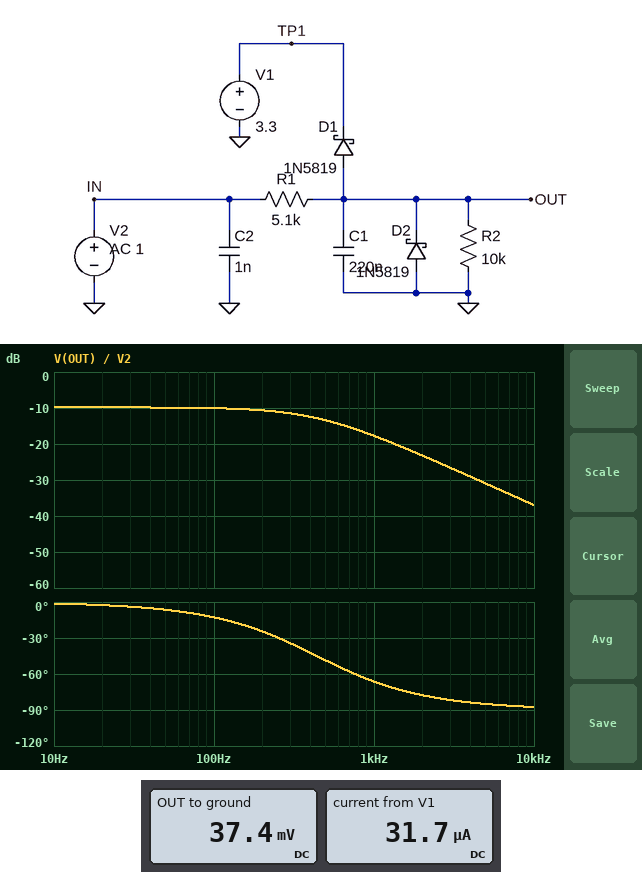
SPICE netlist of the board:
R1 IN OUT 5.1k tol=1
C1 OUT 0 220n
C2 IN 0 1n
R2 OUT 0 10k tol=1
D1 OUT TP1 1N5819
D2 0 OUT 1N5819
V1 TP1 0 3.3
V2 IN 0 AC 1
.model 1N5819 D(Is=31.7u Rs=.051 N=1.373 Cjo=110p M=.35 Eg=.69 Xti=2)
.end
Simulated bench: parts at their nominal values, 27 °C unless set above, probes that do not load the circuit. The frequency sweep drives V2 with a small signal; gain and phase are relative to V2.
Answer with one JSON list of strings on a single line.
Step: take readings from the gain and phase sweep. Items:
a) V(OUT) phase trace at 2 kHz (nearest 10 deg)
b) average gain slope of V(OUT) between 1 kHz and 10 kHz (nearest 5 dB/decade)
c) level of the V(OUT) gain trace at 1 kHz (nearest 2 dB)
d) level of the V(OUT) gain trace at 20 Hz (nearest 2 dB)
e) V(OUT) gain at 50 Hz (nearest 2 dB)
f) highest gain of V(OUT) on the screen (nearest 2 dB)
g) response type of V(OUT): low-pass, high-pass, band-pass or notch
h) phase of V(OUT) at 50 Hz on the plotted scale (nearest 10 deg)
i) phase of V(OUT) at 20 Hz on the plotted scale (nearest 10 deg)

["-80 deg", "-20 dB/decade", "-18 dB", "-10 dB", "-10 dB", "-10 dB", "low-pass", "-10 deg", "0 deg"]
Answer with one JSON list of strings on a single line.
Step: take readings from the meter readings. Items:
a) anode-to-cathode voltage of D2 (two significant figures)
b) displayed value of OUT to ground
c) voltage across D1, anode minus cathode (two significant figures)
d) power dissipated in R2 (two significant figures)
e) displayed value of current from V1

["-37 mV", "37.4 mV", "-3.3 V", "140 nW", "31.7 µA"]
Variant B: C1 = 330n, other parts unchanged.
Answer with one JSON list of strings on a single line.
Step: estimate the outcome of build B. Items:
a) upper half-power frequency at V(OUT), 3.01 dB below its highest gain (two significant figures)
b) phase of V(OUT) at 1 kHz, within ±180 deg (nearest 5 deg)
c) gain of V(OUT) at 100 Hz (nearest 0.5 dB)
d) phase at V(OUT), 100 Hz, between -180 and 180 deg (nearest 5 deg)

["290 Hz", "-75 deg", "-10.5 dB", "-20 deg"]
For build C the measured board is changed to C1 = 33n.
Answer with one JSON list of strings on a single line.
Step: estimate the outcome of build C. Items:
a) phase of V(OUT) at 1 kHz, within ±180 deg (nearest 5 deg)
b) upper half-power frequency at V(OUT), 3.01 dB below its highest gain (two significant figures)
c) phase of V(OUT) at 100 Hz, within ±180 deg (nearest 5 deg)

["-20 deg", "2.9 kHz", "0 deg"]
